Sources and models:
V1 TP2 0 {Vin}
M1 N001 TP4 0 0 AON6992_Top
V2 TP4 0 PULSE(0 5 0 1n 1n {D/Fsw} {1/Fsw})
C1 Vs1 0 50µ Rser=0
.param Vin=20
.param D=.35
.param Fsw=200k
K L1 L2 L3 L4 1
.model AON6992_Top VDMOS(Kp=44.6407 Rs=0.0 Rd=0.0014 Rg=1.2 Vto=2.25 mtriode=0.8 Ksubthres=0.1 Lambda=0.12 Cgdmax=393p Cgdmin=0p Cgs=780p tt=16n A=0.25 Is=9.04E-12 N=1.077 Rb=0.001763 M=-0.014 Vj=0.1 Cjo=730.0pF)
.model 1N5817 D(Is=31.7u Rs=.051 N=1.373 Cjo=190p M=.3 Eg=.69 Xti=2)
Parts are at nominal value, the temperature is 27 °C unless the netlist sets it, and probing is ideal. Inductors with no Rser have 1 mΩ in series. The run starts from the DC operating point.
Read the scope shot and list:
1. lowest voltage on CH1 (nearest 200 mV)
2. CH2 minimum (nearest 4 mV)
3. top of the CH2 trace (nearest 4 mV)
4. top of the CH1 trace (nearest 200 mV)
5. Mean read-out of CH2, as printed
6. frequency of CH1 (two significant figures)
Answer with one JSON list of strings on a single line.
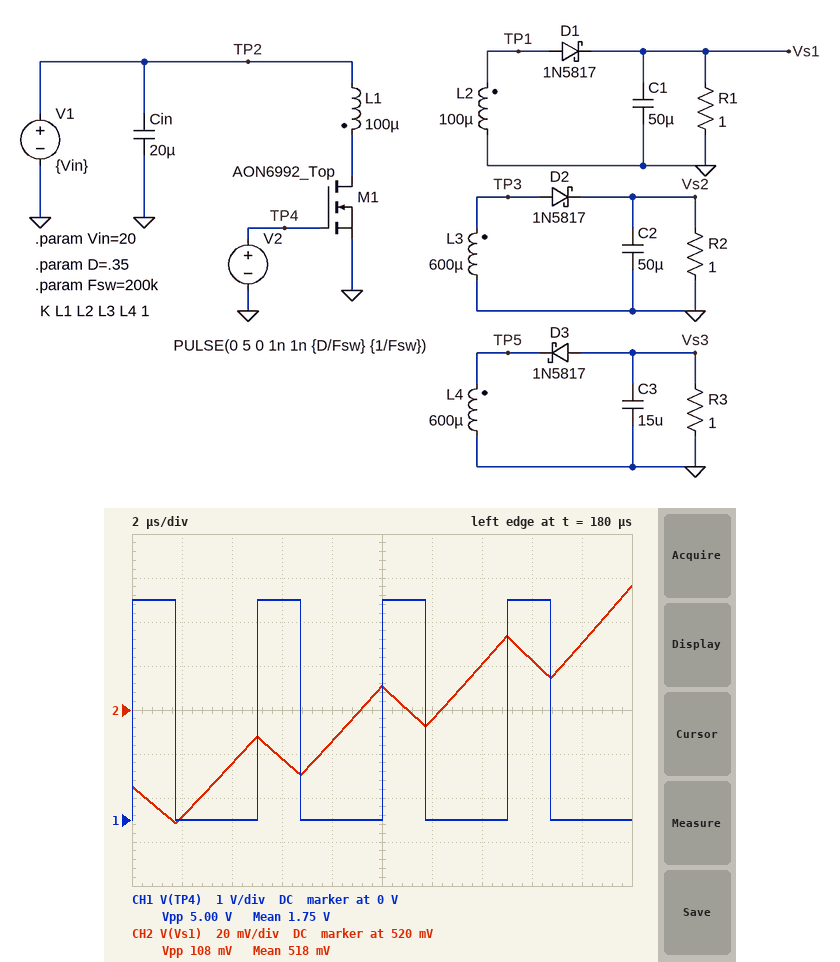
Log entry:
["0 V", "468 mV", "576 mV", "5.0 V", "518 mV", "200 kHz"]
